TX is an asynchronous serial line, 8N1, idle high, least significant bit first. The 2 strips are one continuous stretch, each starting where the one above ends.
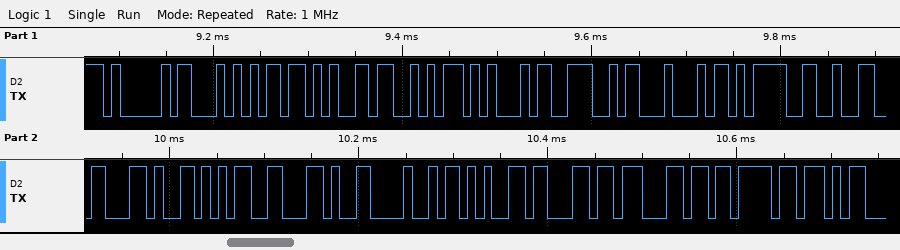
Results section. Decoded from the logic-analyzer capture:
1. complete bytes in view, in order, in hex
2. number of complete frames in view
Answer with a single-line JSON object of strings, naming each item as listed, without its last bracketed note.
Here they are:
{"complete bytes in view, in order, in hex": "0x41 0x54 0x2B 0x53 0x45 0x4E 0x44 0x3D 0x32 0x2C 0x35 0x2C 0x48 0x65 0x6C 0x6C 0x6F", "number of complete frames in view": "17"}
